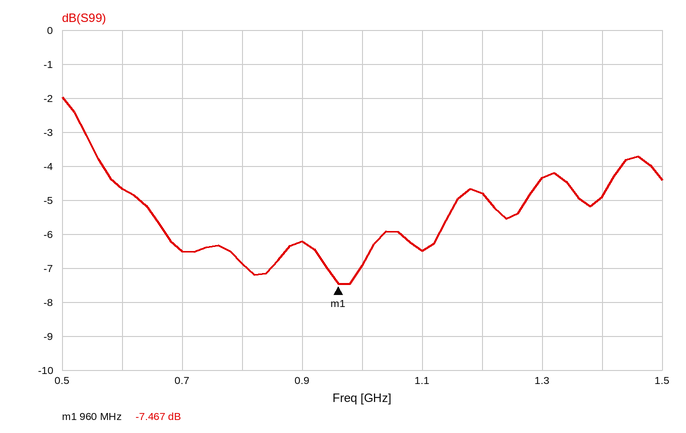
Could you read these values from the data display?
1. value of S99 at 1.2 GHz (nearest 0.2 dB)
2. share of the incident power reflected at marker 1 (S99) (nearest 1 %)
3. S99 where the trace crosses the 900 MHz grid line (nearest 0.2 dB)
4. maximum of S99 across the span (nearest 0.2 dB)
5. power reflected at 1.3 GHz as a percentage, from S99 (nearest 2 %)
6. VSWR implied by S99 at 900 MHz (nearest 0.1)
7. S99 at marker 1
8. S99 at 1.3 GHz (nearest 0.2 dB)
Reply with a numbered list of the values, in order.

1. -4.8 dB
2. 18 %
3. -6.2 dB
4. -2.0 dB
5. 36 %
6. 2.9
7. -7.467 dB
8. -4.4 dB
